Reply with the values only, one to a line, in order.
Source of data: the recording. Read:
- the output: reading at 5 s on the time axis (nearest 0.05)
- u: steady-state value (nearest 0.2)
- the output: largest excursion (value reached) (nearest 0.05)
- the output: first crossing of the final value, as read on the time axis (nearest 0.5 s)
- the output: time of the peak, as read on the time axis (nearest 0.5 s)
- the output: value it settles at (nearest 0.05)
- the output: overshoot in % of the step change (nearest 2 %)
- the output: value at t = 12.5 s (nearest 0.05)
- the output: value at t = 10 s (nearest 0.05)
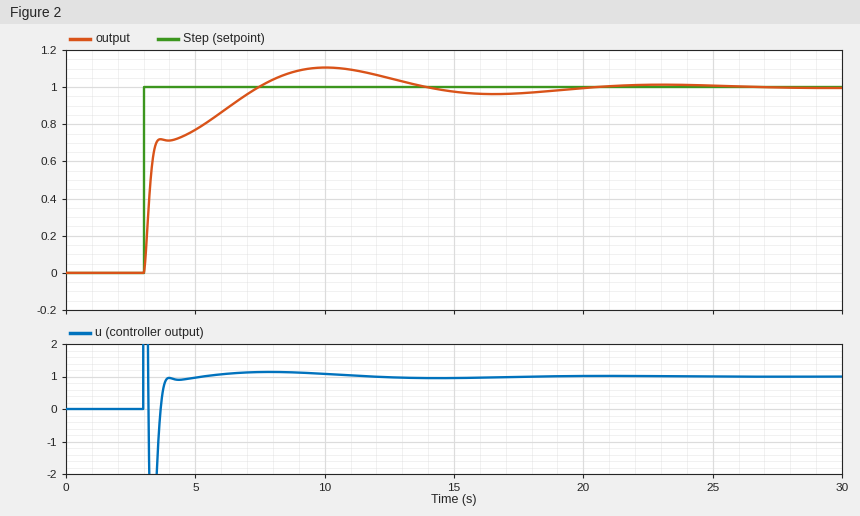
0.75
1.0
1.10
7.5 s
10.0 s
1.00
10 %
1.05
1.10
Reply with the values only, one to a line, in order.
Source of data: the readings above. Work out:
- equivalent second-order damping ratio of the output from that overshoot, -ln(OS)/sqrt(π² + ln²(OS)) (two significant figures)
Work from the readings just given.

0.59
